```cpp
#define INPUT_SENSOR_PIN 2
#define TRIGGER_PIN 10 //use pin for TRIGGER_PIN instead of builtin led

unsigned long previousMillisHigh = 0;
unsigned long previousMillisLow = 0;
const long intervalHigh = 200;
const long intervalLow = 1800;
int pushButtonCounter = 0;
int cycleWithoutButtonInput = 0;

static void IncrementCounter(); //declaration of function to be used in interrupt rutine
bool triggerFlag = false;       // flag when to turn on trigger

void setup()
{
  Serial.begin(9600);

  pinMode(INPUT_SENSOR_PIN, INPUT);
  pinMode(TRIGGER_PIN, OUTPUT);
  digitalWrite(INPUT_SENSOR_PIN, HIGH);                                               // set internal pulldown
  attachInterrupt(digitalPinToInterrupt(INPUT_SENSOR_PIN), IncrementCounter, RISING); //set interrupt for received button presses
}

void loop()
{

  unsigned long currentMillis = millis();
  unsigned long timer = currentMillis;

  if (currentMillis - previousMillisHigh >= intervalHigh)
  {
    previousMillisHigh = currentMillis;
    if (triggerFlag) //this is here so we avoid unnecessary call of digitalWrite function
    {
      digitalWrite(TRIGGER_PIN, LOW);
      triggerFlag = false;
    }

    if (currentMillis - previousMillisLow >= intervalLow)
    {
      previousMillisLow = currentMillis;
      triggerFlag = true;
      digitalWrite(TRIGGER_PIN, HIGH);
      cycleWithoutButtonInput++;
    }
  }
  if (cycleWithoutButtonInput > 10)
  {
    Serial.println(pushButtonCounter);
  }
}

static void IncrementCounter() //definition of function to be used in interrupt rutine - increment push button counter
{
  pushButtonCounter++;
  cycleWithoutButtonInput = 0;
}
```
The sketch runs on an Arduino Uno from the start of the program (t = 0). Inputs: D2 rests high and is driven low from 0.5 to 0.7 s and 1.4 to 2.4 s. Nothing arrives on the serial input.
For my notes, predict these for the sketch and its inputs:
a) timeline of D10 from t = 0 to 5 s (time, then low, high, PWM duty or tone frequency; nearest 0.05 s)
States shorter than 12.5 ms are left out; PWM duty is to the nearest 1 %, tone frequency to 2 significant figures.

0 s low; 1.8 s high; 2 s low; 3.6 s high; 3.8 s low
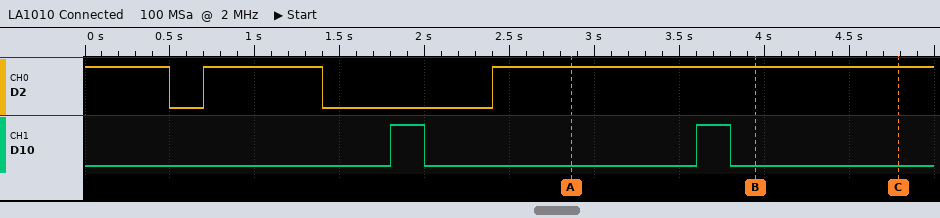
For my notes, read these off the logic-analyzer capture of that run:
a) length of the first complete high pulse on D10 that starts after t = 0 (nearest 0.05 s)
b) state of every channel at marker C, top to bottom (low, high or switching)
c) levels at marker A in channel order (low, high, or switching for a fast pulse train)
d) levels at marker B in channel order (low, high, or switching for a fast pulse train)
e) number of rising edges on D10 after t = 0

0.20 s
D2 high, D10 low
D2 high, D10 low
D2 high, D10 low
2
